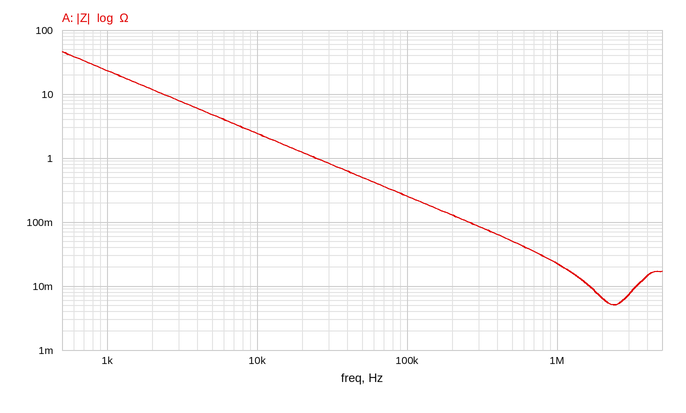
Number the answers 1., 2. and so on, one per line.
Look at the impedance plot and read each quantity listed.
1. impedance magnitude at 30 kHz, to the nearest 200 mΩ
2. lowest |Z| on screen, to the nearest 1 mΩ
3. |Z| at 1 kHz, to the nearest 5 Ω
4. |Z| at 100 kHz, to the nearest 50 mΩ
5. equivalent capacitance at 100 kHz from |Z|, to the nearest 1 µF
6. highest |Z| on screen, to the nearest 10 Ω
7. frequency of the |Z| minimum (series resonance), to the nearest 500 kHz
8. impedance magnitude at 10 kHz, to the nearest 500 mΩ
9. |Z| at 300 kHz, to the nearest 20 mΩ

1. 800 mΩ
2. 5 mΩ
3. 25 Ω
4. 250 mΩ
5. 6 µF
6. 50 Ω
7. 2.5 MHz
8. 2.5 Ω
9. 80 mΩ
